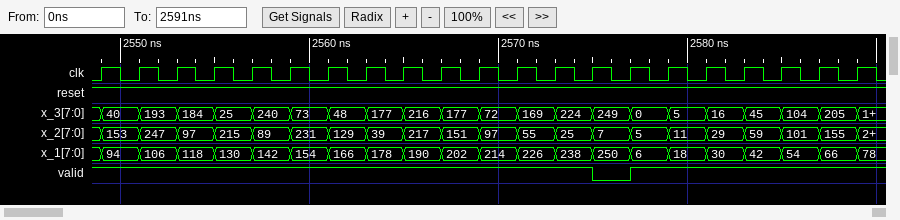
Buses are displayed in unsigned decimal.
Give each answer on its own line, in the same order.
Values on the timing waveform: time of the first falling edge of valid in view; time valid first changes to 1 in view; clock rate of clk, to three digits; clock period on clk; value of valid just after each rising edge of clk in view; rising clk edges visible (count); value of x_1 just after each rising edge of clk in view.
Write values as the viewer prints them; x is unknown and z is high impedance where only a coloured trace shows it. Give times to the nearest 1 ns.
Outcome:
2575 ns
2577 ns
500 MHz
2 ns
1 1 1 1 1 1 1 1 1 1 1 1 1 0 1 1 1 1 1 1 1
21
94, 106, 118, 130, 142, 154, 166, 178, 190, 202, 214, 226, 238, 250, 6, 18, 30, 42, 54, 66, 78
